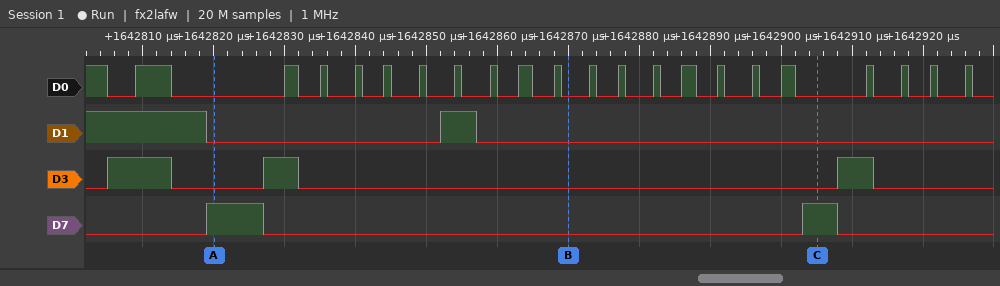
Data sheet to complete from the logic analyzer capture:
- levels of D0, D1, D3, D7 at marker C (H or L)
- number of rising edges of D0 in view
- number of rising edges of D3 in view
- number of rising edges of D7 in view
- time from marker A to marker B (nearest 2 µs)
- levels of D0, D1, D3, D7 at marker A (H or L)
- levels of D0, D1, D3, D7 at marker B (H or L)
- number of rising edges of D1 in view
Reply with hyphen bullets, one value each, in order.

- D0=L, D1=L, D3=L, D7=H
- 21
- 3
- 2
- 50 µs
- D0=L, D1=L, D3=L, D7=H
- D0=L, D1=L, D3=L, D7=L
- 1
